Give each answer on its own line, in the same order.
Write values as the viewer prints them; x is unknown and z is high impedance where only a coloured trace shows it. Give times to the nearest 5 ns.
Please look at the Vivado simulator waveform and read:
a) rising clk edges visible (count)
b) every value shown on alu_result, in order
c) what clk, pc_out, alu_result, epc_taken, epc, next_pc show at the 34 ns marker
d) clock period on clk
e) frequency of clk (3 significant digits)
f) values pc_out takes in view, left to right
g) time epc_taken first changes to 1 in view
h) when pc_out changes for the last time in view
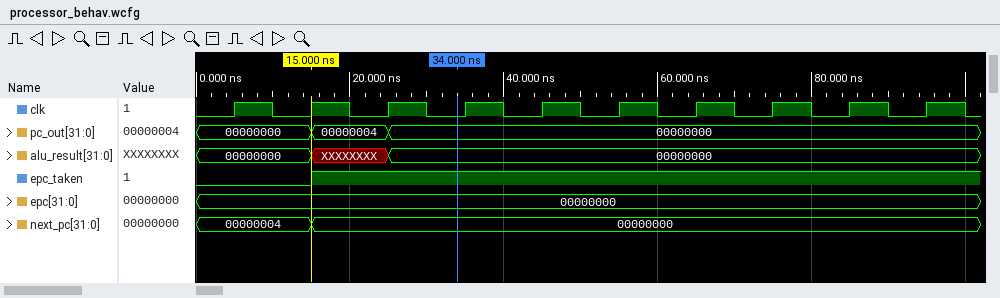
10
00000000, XXXXXXXX, 00000000
clk=0, pc_out=00000000, alu_result=00000000, epc_taken=1, epc=00000000, next_pc=00000000
10 ns
100 MHz
00000000, 00000004, 00000000
15 ns
25 ns
